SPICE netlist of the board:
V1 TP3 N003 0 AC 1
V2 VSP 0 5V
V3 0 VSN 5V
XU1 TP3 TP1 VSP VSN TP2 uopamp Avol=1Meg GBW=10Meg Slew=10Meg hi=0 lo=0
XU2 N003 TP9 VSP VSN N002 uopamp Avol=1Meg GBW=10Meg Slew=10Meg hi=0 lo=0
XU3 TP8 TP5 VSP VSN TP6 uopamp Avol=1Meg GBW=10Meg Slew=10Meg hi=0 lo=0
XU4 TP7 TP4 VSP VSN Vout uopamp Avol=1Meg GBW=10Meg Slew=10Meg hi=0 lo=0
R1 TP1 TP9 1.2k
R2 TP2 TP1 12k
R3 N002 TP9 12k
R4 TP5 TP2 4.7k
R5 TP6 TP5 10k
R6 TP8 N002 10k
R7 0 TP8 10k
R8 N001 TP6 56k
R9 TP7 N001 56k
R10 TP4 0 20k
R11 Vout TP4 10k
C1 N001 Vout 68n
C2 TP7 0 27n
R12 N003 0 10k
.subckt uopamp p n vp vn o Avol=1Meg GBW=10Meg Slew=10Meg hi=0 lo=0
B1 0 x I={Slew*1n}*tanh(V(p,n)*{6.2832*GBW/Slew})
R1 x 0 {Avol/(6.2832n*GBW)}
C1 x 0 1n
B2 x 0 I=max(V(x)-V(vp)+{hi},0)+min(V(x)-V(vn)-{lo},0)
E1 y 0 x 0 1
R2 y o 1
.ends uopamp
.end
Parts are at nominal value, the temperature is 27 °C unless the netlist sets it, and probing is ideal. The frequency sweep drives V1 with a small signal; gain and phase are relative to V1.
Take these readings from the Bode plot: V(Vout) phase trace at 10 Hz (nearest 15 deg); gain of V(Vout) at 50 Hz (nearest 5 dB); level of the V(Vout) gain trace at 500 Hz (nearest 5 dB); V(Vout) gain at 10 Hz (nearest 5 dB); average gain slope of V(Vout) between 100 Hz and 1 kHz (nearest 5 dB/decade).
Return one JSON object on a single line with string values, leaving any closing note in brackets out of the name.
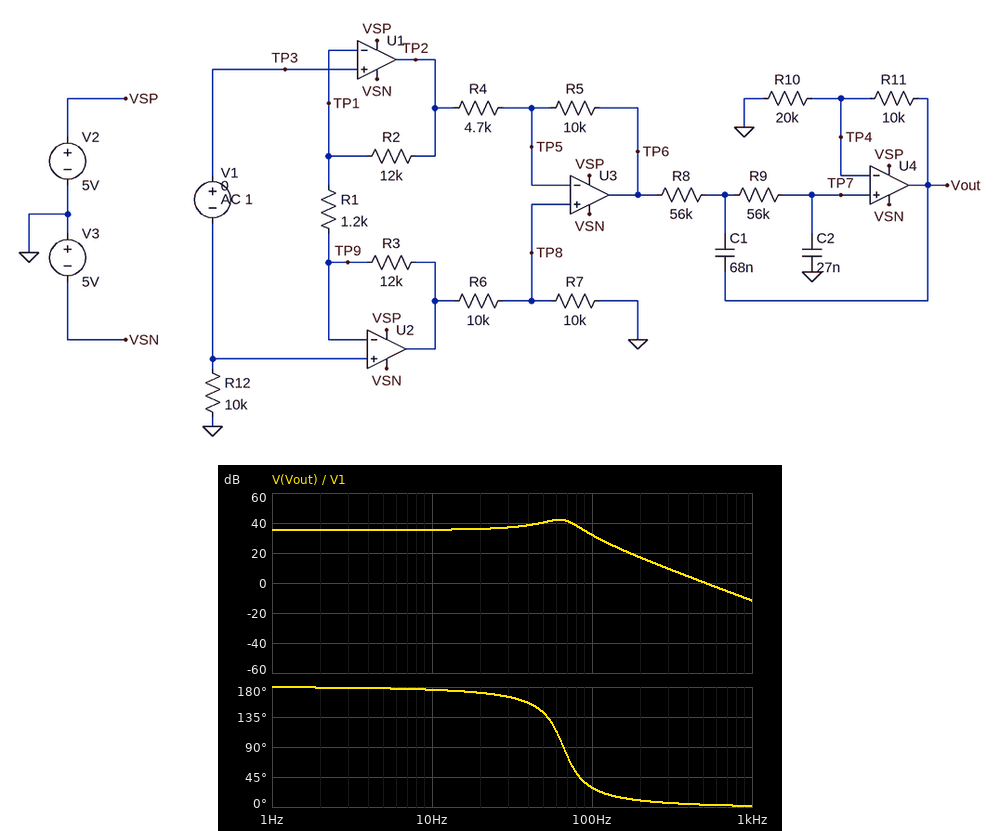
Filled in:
{"V(Vout) phase trace at 10 Hz": "180 deg", "gain of V(Vout) at 50 Hz": "40 dB", "level of the V(Vout) gain trace at 500 Hz": "0 dB", "V(Vout) gain at 10 Hz": "35 dB", "average gain slope of V(Vout) between 100 Hz and 1 kHz": "-45 dB/decade"}
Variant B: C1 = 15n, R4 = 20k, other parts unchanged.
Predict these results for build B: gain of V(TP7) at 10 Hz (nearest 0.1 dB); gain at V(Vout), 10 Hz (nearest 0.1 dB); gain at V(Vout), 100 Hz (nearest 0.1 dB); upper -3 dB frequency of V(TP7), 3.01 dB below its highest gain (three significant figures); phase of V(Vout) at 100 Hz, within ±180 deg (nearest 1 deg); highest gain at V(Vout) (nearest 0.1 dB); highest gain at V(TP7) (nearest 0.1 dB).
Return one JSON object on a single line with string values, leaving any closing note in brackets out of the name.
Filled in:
{"gain of V(TP7) at 10 Hz": "22.2 dB", "gain at V(Vout), 10 Hz": "25.7 dB", "gain at V(Vout), 100 Hz": "21.1 dB", "upper -3 dB frequency of V(TP7), 3.01 dB below its highest gain": "74.3 Hz", "phase of V(Vout) at 100 Hz, within ±180 deg": "107 deg", "highest gain at V(Vout)": "25.8 dB", "highest gain at V(TP7)": "22.3 dB"}
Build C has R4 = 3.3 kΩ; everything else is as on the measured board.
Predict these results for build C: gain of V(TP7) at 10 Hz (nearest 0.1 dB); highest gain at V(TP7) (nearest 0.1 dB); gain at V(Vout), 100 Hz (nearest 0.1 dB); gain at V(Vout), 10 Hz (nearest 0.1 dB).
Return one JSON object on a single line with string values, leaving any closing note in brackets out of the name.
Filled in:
{"gain of V(TP7) at 10 Hz": "34.7 dB", "highest gain at V(TP7)": "41.4 dB", "gain at V(Vout), 100 Hz": "34.8 dB", "gain at V(Vout), 10 Hz": "38.3 dB"}
